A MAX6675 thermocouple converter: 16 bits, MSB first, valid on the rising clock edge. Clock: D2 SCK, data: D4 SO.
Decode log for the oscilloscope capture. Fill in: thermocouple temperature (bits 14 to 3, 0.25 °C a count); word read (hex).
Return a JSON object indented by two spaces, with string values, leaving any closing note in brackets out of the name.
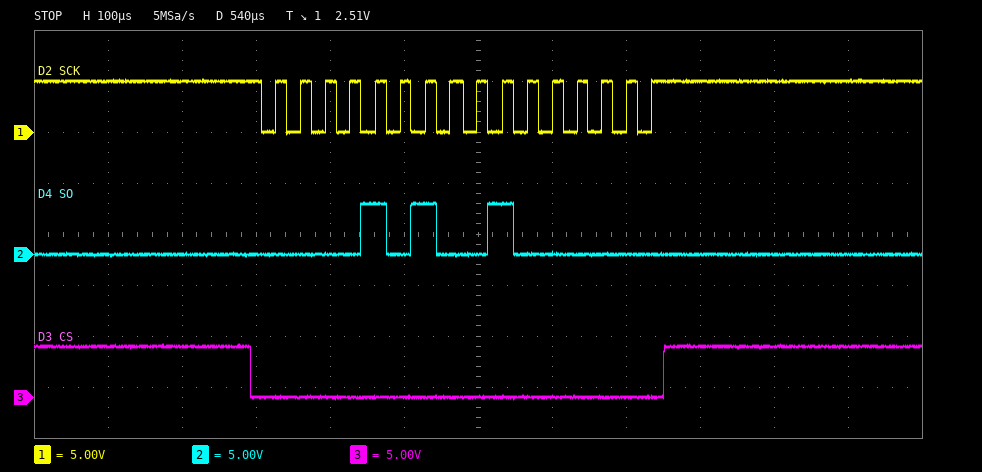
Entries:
{
  "thermocouple temperature": "82.00 °C",
  "word read": "0x0A40"
}
